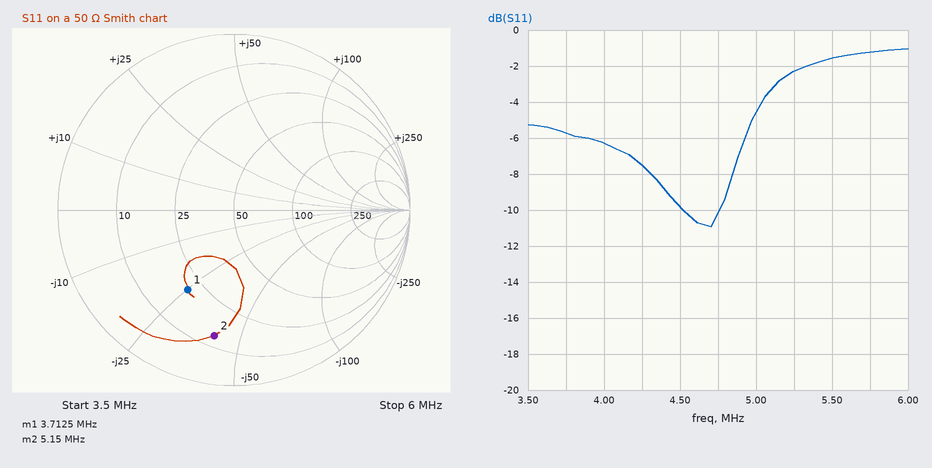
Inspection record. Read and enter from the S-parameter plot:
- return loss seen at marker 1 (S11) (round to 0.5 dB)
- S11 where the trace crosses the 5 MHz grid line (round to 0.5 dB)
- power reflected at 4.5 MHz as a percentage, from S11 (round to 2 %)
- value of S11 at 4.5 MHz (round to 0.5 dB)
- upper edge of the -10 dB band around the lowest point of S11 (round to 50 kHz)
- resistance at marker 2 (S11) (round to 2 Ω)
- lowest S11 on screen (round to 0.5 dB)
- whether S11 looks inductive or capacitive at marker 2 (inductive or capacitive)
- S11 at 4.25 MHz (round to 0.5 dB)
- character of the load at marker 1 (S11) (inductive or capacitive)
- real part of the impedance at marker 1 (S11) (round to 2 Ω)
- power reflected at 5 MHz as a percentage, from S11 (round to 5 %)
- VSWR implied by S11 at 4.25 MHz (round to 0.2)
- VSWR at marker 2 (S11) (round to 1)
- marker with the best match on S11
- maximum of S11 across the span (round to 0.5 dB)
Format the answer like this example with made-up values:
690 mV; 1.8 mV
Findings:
5.5 dB; -4.5 dB; 10 %; -10.0 dB; 4.75 MHz; 14 Ω; -11.0 dB; capacitive; -7.5 dB; capacitive; 20 Ω; 35 %; 2.4; 6; marker 1; -1.0 dB
